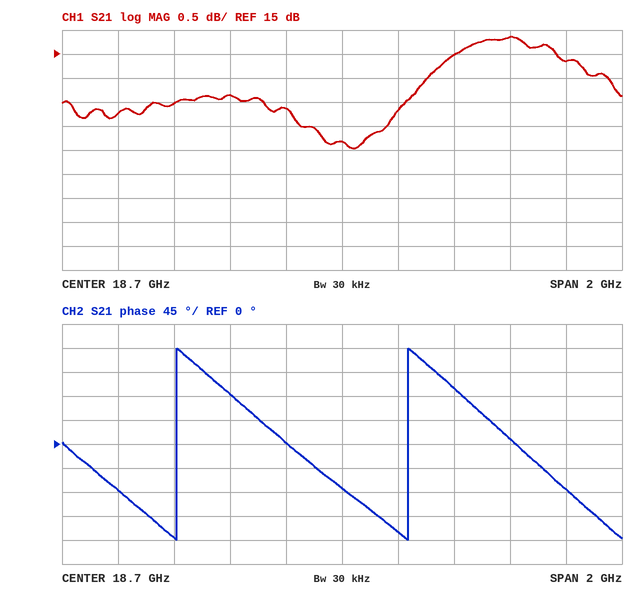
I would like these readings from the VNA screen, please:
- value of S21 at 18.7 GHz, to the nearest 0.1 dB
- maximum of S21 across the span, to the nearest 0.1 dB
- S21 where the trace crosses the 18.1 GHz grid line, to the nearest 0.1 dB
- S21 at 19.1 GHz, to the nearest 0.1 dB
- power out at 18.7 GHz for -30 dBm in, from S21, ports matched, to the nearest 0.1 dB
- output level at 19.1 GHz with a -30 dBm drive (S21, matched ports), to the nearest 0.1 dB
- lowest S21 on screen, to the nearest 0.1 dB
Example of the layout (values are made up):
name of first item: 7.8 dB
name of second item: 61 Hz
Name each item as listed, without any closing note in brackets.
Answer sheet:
value of S21 at 18.7 GHz, to the nearest 0.1 dB: 13.2 dB
maximum of S21 across the span, to the nearest 0.1 dB: 15.4 dB
S21 where the trace crosses the 18.1 GHz grid line, to the nearest 0.1 dB: 14.0 dB
S21 at 19.1 GHz, to the nearest 0.1 dB: 15.0 dB
power out at 18.7 GHz for -30 dBm in, from S21, ports matched, to the nearest 0.1 dB: -16.8 dBm
output level at 19.1 GHz with a -30 dBm drive (S21, matched ports), to the nearest 0.1 dB: -15.0 dBm
lowest S21 on screen, to the nearest 0.1 dB: 13.0 dB
